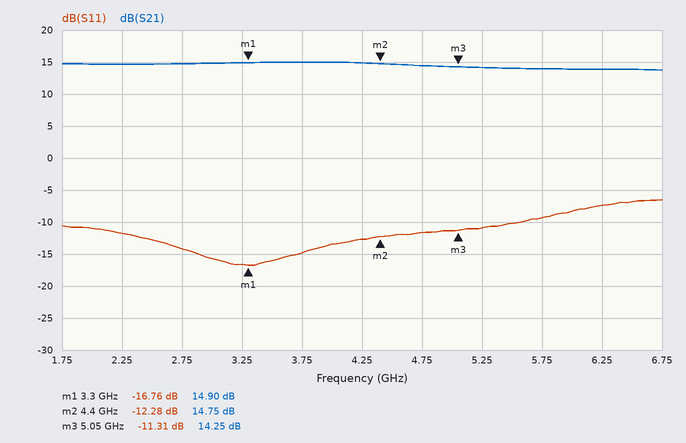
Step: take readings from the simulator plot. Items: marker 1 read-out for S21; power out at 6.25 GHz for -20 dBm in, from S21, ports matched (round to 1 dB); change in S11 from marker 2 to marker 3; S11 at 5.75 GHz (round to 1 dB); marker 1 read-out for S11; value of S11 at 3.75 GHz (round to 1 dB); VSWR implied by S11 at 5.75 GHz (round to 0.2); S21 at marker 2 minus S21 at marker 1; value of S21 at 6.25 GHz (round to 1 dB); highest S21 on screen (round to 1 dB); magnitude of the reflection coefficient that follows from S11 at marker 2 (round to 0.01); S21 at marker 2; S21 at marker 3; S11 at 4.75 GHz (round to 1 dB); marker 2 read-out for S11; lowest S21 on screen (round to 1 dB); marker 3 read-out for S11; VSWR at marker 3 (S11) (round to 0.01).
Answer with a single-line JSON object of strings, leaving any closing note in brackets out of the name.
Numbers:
{"marker 1 read-out for S21": "14.90 dB", "power out at 6.25 GHz for -20 dBm in, from S21, ports matched": "-6 dBm", "change in S11 from marker 2 to marker 3": "0.97 dB", "S11 at 5.75 GHz": "-9 dB", "marker 1 read-out for S11": "-16.76 dB", "value of S11 at 3.75 GHz": "-15 dB", "VSWR implied by S11 at 5.75 GHz": "2.0", "S21 at marker 2 minus S21 at marker 1": "-0.15 dB", "value of S21 at 6.25 GHz": "14 dB", "highest S21 on screen": "15 dB", "magnitude of the reflection coefficient that follows from S11 at marker 2": "0.24", "S21 at marker 2": "14.75 dB", "S21 at marker 3": "14.25 dB", "S11 at 4.75 GHz": "-12 dB", "marker 2 read-out for S11": "-12.28 dB", "lowest S21 on screen": "14 dB", "marker 3 read-out for S11": "-11.31 dB", "VSWR at marker 3 (S11)": "1.75"}
